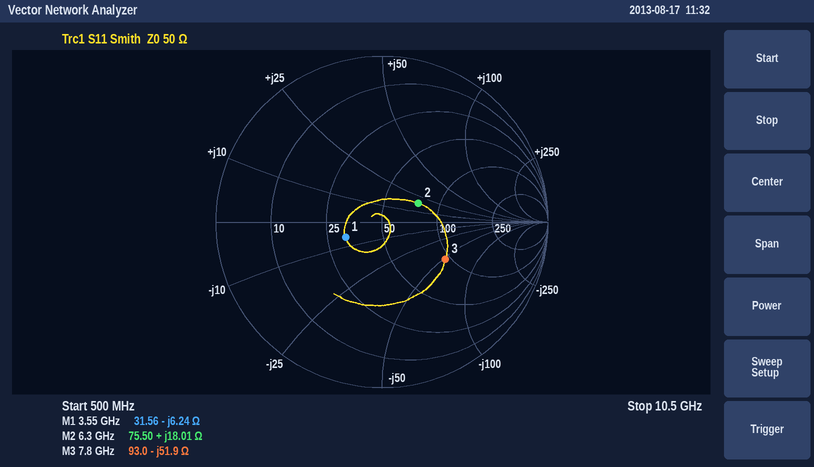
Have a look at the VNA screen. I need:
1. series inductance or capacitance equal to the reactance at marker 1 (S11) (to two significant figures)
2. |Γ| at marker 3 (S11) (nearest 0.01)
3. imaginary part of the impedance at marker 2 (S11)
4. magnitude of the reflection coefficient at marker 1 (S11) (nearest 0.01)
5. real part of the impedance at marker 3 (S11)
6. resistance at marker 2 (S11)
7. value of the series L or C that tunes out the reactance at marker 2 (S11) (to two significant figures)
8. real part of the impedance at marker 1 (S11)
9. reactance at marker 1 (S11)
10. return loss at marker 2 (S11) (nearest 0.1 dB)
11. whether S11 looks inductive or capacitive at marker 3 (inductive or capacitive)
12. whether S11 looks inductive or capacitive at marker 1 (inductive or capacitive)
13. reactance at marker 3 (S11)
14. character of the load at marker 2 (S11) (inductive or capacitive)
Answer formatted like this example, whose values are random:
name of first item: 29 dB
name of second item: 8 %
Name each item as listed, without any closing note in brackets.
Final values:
series inductance or capacitance equal to the reactance at marker 1 (S11): 7.2 pF
|Γ| at marker 3 (S11): 0.44
imaginary part of the impedance at marker 2: +18.01 Ω
magnitude of the reflection coefficient at marker 1 (S11): 0.24
real part of the impedance at marker 3: 93.0 Ω
resistance at marker 2: 75.50 Ω
value of the series L or C that tunes out the reactance at marker 2 (S11): 1.4 pF
real part of the impedance at marker 1: 31.56 Ω
reactance at marker 1: -6.24 Ω
return loss at marker 2 (S11): 12.2 dB
whether S11 looks inductive or capacitive at marker 3: capacitive
whether S11 looks inductive or capacitive at marker 1: capacitive
reactance at marker 3: -51.9 Ω
character of the load at marker 2 (S11): inductive
